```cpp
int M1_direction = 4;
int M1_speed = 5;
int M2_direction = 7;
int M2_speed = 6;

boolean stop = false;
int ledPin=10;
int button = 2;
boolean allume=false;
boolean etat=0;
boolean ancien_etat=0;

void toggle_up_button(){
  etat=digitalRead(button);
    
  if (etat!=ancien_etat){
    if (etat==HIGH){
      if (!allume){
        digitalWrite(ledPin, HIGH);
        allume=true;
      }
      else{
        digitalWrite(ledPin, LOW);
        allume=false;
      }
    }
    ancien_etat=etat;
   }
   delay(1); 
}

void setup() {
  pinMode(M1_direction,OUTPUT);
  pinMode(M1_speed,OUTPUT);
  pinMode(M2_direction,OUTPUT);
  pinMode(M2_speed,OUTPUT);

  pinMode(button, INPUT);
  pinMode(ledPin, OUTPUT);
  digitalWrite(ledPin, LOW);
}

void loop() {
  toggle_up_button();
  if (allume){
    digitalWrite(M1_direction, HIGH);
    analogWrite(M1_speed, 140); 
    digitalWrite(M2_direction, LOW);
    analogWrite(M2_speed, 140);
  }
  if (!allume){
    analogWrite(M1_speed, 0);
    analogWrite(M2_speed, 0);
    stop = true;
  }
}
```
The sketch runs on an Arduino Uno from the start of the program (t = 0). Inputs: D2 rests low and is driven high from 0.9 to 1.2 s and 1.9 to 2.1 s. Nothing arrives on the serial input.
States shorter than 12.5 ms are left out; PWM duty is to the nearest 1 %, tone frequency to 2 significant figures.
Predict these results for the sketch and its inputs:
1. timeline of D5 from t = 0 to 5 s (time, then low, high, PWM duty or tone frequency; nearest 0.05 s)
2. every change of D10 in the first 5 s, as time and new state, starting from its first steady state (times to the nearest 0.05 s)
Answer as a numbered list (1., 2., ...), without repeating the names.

1. 0 s low; 0.9 s PWM 55 %; 1.9 s low
2. 0 s low; 0.9 s high; 1.9 s low
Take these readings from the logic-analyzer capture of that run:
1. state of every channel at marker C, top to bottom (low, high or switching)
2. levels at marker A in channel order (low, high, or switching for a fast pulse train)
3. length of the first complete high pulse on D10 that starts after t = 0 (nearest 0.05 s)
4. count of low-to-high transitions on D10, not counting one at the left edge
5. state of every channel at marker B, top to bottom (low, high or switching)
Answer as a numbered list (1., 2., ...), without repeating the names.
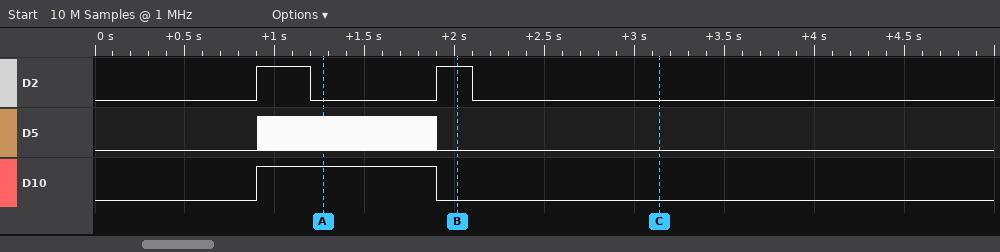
1. D2 low, D5 low, D10 low
2. D2 low, D5 switching, D10 high
3. 1.00 s
4. 1
5. D2 high, D5 low, D10 low
